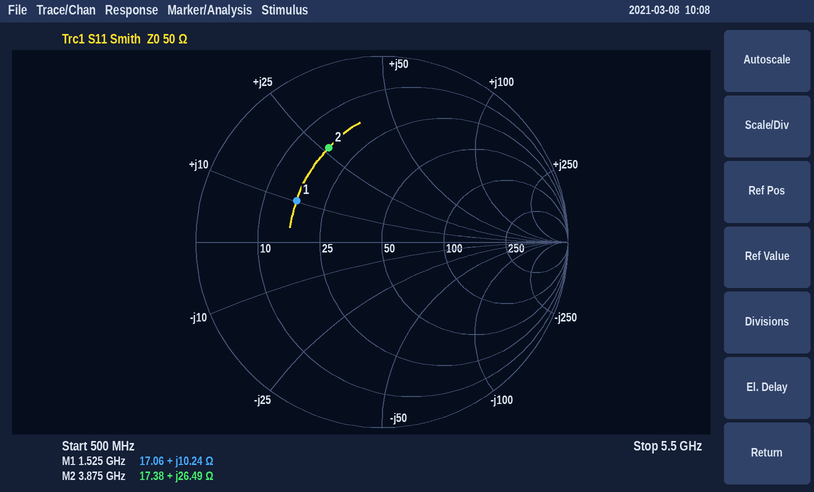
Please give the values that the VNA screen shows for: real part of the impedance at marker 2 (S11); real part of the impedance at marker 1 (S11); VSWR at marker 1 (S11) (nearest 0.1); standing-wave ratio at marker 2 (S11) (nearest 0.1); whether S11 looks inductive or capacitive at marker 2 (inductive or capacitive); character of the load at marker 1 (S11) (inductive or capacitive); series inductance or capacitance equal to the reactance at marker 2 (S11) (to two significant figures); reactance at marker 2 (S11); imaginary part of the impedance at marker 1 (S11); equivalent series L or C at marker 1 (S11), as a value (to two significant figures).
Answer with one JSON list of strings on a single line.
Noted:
["17.38 Ω", "17.06 Ω", "3.1", "3.8", "inductive", "inductive", "1.1 nH", "+26.49 Ω", "+10.24 Ω", "1.1 nH"]
